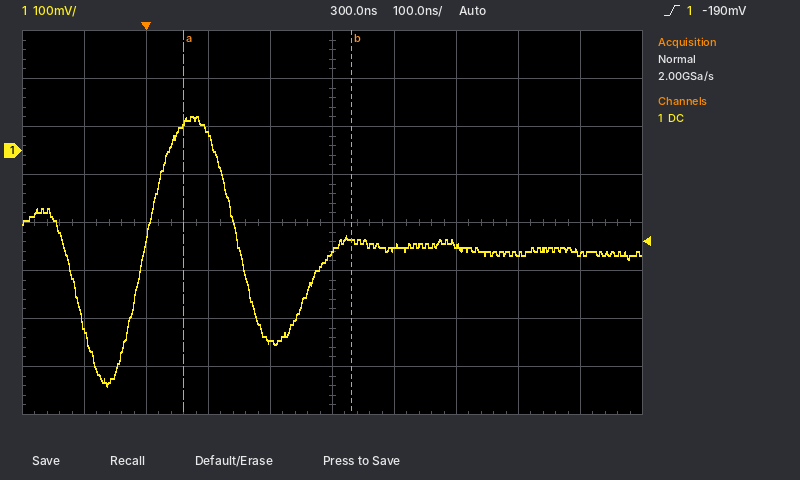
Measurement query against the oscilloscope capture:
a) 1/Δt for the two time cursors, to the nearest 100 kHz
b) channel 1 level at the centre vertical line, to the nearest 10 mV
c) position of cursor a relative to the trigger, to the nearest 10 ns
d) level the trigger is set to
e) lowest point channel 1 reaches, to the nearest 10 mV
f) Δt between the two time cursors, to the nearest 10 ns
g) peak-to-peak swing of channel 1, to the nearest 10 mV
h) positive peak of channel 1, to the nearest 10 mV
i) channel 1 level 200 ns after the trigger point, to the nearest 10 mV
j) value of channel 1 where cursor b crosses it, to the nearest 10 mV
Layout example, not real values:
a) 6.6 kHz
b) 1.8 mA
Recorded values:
a) 3.7 MHz
b) -210 mV
c) +60 ns
d) -190 mV
e) -490 mV
f) 270 ns
g) 560 mV
h) 70 mV
i) -400 mV
j) -190 mV
